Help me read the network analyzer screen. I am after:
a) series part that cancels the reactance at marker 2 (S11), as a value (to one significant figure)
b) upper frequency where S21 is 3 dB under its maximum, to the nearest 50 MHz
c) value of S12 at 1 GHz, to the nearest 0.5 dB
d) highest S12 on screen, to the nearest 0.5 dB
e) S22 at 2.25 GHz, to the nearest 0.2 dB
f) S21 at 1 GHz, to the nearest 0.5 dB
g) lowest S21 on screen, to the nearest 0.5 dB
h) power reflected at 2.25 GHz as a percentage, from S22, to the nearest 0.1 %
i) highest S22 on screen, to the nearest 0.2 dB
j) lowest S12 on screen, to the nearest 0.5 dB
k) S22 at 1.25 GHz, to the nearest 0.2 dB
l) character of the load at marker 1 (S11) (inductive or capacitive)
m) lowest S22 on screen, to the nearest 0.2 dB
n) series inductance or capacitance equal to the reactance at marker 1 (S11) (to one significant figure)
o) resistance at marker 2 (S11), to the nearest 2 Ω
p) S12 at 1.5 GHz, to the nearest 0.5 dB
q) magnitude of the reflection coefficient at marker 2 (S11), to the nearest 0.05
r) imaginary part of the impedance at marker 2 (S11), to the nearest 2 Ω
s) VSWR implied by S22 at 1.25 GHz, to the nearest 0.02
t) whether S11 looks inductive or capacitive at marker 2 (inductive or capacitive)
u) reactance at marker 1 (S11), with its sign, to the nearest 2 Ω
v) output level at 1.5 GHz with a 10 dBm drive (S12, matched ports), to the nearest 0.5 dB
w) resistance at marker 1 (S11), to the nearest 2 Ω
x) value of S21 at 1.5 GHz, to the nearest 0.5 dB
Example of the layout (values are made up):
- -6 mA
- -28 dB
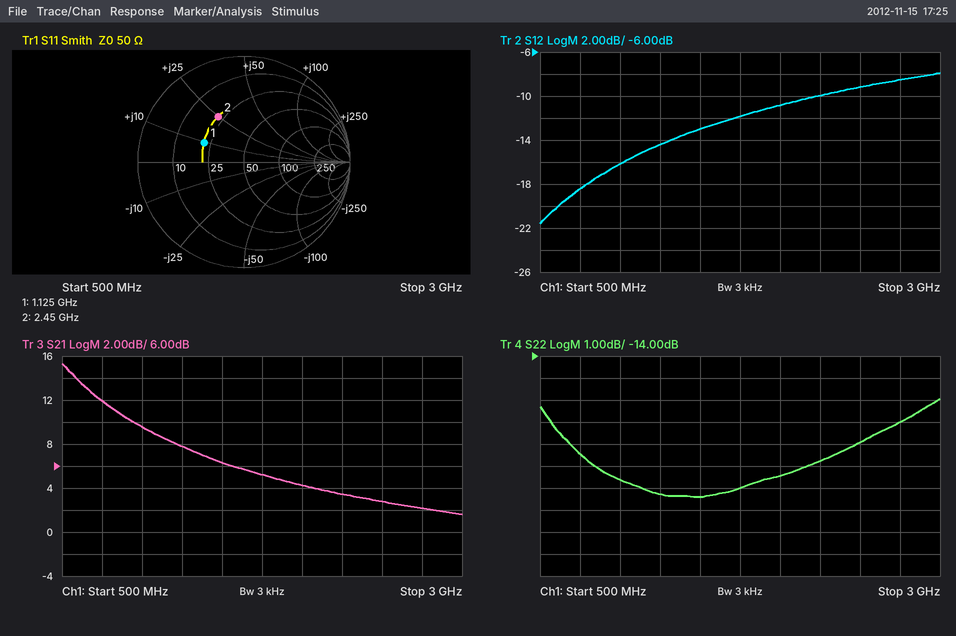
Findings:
- 3 pF
- 700 MHz
- -16.0 dB
- -8.0 dB
- -18.8 dB
- 9.5 dB
- 1.5 dB
- 1.3 %
- -16.0 dB
- -21.5 dB
- -20.2 dB
- inductive
- -20.4 dB
- 1 nH
- 22 Ω
- -13.0 dB
- 0.50
- +24 Ω
- 1.22
- inductive
- +10 Ω
- -3.0 dBm
- 22 Ω
- 6.5 dB
